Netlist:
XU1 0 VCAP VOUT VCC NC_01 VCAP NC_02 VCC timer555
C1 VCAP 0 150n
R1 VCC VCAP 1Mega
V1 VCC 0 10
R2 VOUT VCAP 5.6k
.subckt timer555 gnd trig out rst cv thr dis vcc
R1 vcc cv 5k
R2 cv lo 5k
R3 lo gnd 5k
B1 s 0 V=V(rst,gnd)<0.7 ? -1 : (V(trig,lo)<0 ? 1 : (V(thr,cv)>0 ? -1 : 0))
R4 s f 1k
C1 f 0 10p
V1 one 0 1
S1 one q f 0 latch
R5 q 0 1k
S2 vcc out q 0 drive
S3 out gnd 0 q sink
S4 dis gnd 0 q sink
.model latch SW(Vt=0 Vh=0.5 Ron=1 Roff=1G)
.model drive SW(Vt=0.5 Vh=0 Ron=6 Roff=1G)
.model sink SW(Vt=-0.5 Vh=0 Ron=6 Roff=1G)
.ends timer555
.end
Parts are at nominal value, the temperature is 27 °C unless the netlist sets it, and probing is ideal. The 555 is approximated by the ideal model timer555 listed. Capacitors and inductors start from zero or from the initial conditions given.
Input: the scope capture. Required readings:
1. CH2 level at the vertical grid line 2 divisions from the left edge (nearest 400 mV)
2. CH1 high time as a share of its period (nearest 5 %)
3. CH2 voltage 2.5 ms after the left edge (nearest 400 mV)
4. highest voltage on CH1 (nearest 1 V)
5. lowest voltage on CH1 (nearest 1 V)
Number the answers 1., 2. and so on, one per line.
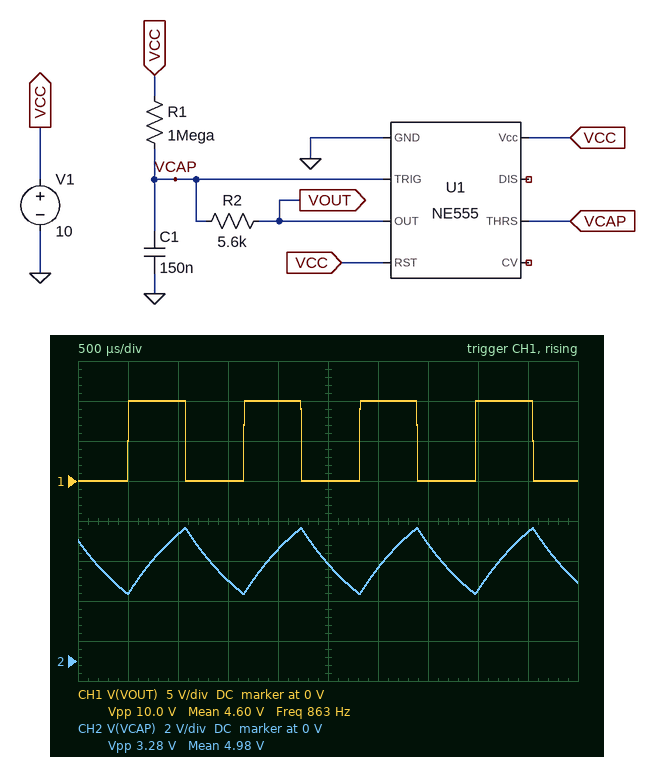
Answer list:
1. 6.4 V
2. 50 %
3. 4.8 V
4. 10 V
5. 0 V
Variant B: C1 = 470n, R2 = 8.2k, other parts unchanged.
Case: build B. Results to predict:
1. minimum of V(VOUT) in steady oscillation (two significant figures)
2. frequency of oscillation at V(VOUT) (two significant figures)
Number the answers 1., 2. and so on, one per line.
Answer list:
1. 2.4 mV
2. 190 Hz
